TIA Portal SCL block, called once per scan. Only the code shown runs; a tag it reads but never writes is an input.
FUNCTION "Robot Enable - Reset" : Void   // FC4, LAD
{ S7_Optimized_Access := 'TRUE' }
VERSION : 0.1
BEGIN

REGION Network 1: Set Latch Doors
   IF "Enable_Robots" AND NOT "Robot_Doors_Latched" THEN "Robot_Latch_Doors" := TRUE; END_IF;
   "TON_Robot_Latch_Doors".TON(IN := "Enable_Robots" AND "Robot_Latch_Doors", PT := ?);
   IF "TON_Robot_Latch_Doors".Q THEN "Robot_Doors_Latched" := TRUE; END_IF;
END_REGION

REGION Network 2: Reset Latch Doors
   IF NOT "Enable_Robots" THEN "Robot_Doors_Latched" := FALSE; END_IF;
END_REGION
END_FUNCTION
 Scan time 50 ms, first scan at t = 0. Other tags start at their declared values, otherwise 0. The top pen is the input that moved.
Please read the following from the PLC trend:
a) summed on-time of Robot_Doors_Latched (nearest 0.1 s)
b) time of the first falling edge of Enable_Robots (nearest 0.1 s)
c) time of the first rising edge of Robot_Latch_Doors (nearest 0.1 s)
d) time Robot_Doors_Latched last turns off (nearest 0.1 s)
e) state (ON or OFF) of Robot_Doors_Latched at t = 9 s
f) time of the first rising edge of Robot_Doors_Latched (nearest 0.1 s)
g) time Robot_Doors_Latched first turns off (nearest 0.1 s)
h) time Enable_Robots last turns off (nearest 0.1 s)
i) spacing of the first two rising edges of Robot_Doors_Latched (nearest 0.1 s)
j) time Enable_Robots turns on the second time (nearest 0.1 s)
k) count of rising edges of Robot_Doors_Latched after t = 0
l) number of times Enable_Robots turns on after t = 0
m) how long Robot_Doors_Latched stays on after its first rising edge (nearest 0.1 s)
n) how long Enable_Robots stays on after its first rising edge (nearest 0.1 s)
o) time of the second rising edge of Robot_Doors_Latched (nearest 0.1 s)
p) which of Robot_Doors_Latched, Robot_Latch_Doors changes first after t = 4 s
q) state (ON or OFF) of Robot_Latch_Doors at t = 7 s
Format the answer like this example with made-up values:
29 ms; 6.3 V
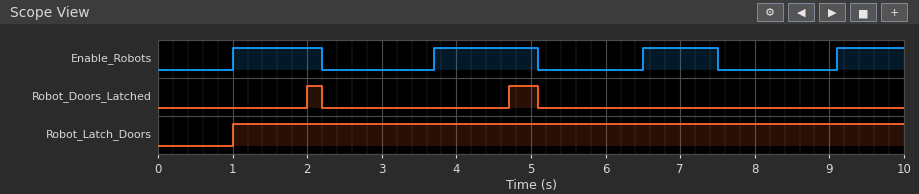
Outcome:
0.6 s; 2.2 s; 1.0 s; 5.1 s; OFF; 2.0 s; 2.2 s; 7.5 s; 2.7 s; 3.7 s; 2; 4; 0.2 s; 1.2 s; 4.7 s; Robot_Doors_Latched; ON
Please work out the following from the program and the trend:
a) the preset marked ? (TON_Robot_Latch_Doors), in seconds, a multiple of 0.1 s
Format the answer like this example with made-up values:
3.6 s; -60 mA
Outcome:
1.0 s
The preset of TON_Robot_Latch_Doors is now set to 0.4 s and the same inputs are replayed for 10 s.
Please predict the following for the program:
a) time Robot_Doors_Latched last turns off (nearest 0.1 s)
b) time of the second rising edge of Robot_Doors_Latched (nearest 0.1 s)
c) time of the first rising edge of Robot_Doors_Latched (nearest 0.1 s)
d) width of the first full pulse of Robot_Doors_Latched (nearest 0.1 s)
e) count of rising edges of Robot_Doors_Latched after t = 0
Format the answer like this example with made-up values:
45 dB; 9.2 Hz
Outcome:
7.5 s; 4.1 s; 1.4 s; 0.8 s; 4
